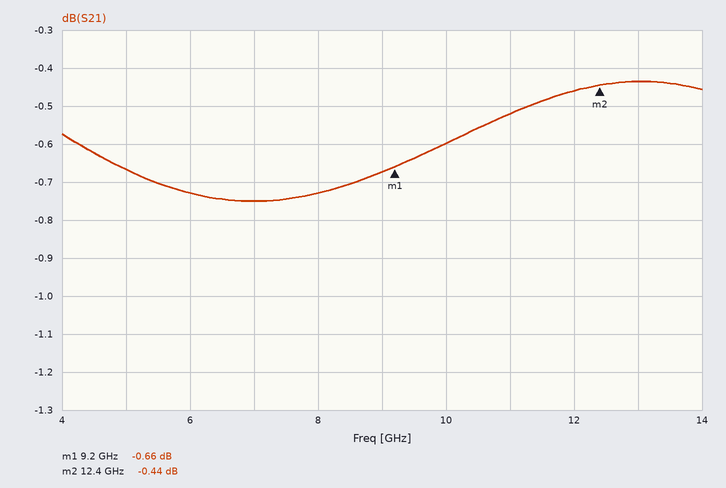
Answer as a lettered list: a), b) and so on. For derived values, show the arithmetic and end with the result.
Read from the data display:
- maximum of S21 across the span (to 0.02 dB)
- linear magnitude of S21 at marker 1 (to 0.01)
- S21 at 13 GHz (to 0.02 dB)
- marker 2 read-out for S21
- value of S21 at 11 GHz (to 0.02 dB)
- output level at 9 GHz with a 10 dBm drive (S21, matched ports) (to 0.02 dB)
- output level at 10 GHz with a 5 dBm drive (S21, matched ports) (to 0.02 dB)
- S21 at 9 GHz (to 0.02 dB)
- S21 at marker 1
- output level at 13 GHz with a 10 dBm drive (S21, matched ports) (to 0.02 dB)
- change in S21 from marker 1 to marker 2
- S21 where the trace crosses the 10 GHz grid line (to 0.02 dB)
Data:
a) -0.44 dB
b) 10^(-0.66/20) ≈ 0.93
c) -0.44 dB
d) -0.44 dB
e) -0.52 dB
f) 10 dBm + (-0.68 dB) = 9.32 dBm
g) 5 dBm + (-0.60 dB) = 4.40 dBm
h) -0.68 dB
i) -0.66 dB
j) 10 dBm + (-0.44 dB) = 9.56 dBm
k) -0.44 − (-0.66) = 0.22 dB
l) -0.60 dB
